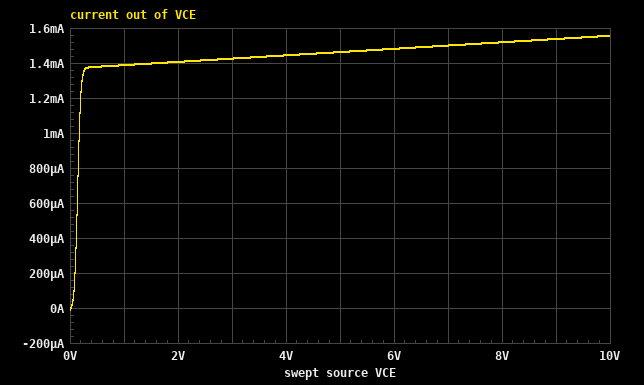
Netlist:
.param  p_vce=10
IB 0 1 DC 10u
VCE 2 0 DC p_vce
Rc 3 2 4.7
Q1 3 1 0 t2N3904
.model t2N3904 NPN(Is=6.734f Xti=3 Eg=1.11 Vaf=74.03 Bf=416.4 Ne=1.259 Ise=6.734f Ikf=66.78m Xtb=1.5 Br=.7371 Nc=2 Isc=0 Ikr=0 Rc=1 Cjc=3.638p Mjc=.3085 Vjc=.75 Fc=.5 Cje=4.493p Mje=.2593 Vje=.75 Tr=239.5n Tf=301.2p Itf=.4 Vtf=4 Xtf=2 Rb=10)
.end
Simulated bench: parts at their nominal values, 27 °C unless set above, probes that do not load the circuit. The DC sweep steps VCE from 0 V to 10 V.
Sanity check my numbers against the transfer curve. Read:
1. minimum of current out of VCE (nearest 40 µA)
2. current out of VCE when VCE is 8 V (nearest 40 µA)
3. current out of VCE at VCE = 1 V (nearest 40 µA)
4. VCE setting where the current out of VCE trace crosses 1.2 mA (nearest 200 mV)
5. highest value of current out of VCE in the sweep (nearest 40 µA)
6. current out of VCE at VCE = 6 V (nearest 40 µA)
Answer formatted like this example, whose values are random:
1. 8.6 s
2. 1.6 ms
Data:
1. 0 A
2. 1.52 mA
3. 1.40 mA
4. 200 mV
5. 1.56 mA
6. 1.48 mA
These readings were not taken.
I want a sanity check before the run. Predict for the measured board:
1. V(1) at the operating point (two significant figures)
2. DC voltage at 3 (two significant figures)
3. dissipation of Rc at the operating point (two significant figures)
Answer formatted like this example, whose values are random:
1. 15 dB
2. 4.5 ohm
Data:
1. 670 mV
2. 10 V
3. 11 µW
